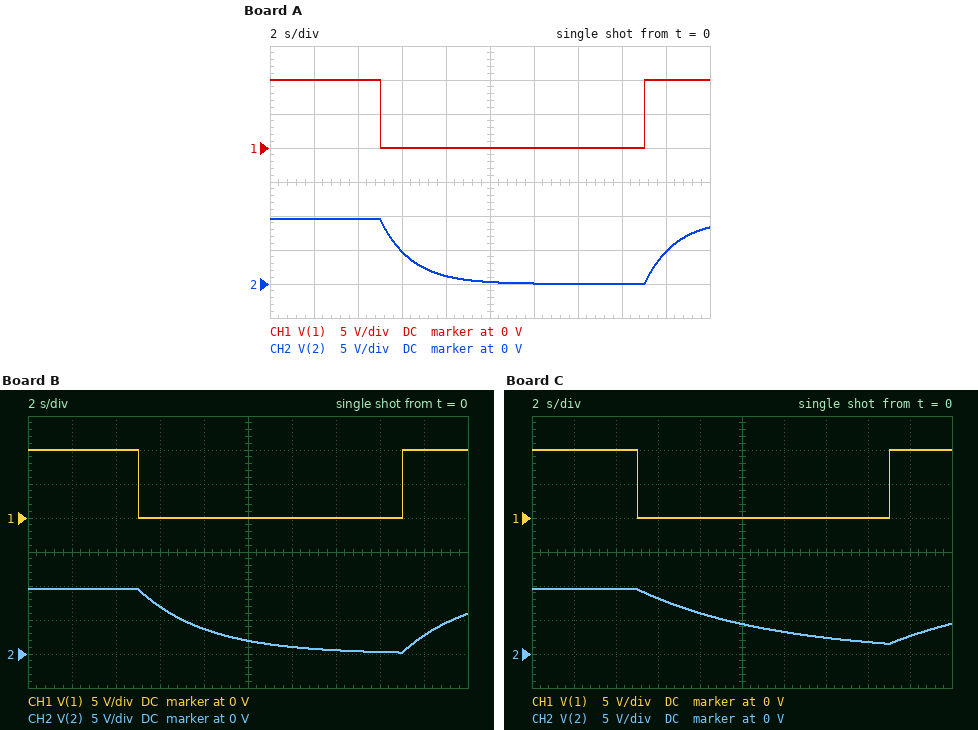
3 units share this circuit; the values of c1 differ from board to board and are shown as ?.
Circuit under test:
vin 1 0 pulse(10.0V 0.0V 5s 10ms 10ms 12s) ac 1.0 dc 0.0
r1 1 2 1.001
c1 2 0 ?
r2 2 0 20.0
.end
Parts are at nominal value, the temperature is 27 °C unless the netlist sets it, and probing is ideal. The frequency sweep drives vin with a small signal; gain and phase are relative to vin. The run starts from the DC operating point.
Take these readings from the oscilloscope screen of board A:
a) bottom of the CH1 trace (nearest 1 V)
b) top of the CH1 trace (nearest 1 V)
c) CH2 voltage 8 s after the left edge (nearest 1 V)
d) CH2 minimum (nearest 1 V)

0 V
10 V
1 V
0 V
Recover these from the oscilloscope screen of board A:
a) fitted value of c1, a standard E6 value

1.5 F
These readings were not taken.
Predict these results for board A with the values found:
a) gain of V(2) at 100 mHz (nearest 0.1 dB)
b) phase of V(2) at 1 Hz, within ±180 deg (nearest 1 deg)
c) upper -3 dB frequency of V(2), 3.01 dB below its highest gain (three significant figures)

-3.0 dB
-84 deg
111 mHz
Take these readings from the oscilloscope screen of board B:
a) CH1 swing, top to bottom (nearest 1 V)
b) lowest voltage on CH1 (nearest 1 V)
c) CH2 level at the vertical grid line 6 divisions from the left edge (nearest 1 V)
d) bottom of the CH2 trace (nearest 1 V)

10 V
0 V
1 V
0 V
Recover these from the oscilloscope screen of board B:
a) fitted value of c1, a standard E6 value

3.3 F
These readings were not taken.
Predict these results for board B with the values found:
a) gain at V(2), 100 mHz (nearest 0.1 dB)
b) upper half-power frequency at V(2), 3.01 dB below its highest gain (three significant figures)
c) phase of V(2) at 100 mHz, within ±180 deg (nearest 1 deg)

-7.3 dB
50.6 mHz
-63 deg
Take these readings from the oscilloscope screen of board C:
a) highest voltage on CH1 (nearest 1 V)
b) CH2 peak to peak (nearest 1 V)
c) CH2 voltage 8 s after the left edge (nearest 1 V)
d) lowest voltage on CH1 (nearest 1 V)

10 V
8 V
6 V
0 V
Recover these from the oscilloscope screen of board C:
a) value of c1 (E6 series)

6.8 F
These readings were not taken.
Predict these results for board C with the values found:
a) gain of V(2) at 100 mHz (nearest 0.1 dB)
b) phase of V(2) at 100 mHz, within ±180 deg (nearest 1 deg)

-12.9 dB
-76 deg
